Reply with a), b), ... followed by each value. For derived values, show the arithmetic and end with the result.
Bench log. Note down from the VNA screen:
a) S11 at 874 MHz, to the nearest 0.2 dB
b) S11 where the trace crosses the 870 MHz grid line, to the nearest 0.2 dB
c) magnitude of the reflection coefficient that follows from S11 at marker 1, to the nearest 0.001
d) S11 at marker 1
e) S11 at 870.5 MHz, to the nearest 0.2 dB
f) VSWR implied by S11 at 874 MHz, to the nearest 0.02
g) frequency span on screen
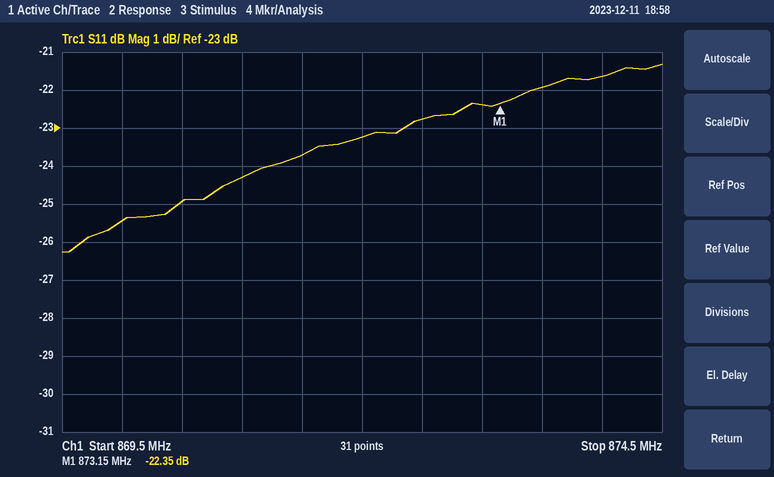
a) -21.6 dB
b) -25.4 dB
c) 10^(-22.35/20) ≈ 0.076
d) -22.35 dB
e) -25.0 dB
f) |Γ| = 10^(-21.6/20) = 0.0832; VSWR = (1 + 0.0832)/(1 − 0.0832) ≈ 1.18
g) 5 MHz
